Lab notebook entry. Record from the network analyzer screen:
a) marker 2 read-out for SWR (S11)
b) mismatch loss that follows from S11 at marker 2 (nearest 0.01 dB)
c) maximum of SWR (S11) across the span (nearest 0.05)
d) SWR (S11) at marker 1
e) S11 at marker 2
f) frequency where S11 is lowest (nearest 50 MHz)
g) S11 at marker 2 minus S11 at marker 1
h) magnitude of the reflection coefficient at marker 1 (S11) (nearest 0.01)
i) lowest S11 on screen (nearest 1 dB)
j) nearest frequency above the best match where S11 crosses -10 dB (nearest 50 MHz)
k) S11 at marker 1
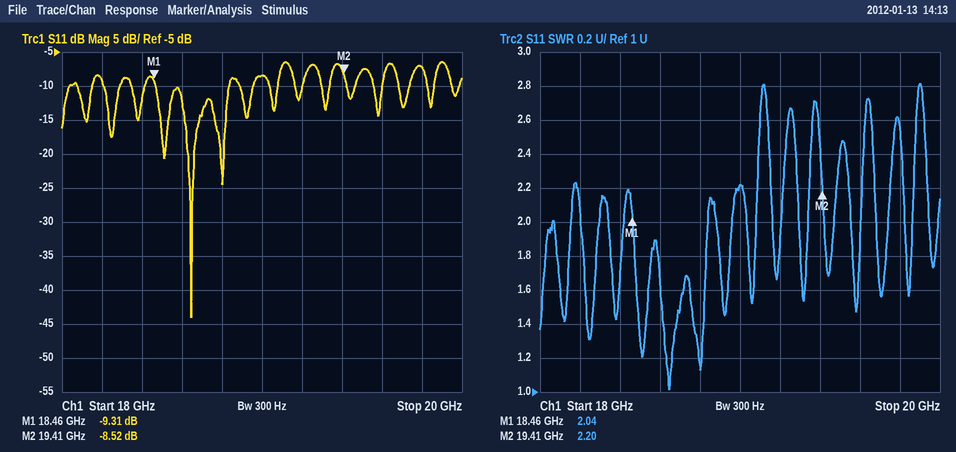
2.20
0.66 dB
2.80
2.04
-8.52 dB
18.65 GHz
0.79 dB
0.34
-44 dB
18.85 GHz
-9.31 dB
